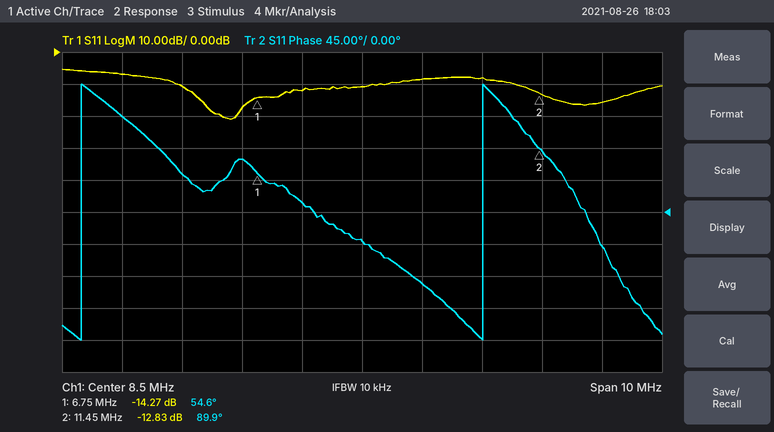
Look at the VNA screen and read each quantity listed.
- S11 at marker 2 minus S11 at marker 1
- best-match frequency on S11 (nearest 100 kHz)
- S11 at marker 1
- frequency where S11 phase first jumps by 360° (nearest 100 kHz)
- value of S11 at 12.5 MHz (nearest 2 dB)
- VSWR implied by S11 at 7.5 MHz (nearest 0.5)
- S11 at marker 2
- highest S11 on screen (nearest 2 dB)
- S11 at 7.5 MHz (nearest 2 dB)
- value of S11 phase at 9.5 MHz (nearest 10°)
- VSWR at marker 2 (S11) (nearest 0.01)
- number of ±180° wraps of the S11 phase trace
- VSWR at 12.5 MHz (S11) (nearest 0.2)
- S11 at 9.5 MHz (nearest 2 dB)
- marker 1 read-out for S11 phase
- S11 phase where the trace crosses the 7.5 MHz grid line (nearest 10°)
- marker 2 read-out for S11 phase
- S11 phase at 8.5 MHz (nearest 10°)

1.44 dB
6.3 MHz
-14.27 dB
3.8 MHz
-16 dB
1.5
-12.83 dB
-6 dB
-12 dB
-100°
1.59
2
1.4
-8 dB
54.6°
10°
89.9°
-40°
